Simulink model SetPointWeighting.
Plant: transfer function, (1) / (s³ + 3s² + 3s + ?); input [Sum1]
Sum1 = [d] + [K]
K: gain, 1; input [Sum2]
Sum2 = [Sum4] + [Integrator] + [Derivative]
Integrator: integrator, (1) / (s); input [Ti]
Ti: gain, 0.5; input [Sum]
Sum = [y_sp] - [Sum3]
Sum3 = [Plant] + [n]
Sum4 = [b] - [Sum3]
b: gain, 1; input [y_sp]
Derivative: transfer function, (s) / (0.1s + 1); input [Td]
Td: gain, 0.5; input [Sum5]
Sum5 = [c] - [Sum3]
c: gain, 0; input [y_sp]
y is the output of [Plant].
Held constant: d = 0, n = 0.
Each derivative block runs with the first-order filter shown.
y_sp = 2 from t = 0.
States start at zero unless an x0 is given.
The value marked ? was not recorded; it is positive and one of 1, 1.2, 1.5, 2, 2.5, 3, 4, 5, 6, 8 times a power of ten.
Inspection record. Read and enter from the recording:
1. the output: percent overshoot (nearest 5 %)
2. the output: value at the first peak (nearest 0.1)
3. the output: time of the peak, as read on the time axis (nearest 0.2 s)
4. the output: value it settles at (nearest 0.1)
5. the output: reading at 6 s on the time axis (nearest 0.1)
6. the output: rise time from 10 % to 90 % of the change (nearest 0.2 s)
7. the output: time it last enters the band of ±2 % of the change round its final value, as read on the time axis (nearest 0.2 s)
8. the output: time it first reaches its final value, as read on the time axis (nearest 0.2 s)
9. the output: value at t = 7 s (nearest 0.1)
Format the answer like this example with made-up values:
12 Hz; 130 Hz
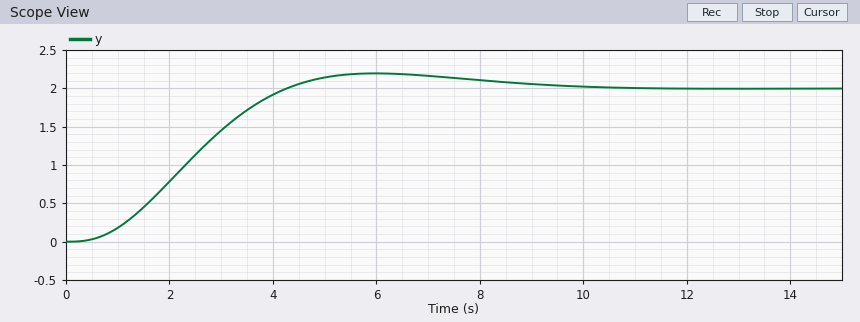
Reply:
10 %; 2.2; 6.0 s; 2.0; 2.2; 2.6 s; 9.4 s; 4.2 s; 2.2
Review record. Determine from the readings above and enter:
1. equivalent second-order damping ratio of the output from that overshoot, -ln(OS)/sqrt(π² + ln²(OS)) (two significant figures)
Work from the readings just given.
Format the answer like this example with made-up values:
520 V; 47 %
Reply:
0.59
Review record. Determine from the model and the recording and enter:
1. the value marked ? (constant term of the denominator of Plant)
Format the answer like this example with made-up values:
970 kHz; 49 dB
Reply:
1
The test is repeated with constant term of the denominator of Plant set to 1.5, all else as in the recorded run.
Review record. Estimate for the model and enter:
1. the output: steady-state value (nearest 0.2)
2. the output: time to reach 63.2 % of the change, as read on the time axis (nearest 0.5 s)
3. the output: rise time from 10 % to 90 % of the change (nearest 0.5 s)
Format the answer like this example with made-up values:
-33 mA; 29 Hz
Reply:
2.0; 3.0 s; 3.5 s
